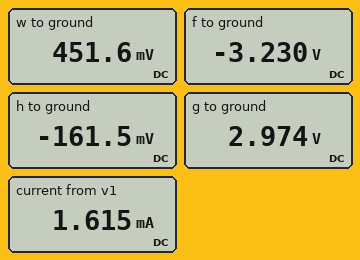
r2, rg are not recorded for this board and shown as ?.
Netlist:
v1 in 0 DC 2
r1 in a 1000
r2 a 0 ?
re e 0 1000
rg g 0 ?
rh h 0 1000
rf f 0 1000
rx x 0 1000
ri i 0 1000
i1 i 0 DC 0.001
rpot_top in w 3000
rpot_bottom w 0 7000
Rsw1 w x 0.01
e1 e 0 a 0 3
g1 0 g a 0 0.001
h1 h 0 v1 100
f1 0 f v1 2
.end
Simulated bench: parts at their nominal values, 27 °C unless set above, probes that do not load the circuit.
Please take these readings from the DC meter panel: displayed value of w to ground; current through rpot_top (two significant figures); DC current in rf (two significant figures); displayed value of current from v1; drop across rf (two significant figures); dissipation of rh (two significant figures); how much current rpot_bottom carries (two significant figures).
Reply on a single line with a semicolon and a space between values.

451.6 mV; 520 µA; 3.2 mA; 1.615 mA; 3.2 V; 26 µW; 65 µA
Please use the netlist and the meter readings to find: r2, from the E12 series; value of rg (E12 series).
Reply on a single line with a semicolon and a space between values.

820 Ω; 3.3 kΩ
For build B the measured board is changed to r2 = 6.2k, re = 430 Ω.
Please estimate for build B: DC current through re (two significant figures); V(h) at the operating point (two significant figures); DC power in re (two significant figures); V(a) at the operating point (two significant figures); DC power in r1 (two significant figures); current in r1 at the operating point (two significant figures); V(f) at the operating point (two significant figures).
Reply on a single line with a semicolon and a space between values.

12 mA; -79 mV; 62 mW; 1.7 V; 77 µW; 280 µA; -1.6 V
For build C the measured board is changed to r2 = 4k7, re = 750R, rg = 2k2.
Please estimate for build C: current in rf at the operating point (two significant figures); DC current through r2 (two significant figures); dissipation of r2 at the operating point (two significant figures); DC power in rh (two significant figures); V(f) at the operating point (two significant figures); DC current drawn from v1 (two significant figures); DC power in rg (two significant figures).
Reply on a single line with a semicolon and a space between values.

1.7 mA; 350 µA; 580 µW; 7.5 µW; -1.7 V; 870 µA; 6.0 mW
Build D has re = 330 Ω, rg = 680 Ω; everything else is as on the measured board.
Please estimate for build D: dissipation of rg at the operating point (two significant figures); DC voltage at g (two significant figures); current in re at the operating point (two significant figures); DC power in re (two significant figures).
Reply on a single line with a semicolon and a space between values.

550 µW; 610 mV; 8.2 mA; 22 mW
